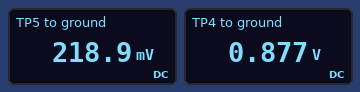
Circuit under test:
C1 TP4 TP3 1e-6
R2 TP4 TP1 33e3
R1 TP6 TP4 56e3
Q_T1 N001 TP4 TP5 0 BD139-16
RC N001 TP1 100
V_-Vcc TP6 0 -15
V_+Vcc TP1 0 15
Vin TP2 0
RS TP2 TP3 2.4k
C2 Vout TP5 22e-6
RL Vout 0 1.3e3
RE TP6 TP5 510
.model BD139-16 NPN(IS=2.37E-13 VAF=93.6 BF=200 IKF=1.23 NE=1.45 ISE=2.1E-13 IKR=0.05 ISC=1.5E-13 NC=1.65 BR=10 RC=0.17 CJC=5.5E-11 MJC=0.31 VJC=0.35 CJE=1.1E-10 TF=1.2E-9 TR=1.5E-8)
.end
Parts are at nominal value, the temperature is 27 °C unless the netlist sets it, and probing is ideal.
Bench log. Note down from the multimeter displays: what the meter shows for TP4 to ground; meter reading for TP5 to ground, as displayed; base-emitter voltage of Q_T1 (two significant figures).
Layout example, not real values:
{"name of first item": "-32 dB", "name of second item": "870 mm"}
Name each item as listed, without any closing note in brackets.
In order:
{"what the meter shows for TP4 to ground": "0.877 V", "meter reading for TP5 to ground, as displayed": "218.9 mV", "base-emitter voltage of Q_T1": "660 mV"}
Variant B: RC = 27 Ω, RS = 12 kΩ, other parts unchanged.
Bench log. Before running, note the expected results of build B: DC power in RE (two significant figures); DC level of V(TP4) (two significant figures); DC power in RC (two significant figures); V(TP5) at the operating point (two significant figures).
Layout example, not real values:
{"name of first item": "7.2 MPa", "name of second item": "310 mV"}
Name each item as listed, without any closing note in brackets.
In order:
{"DC power in RE": "460 mW", "DC level of V(TP4)": "930 mV", "DC power in RC": "24 mW", "V(TP5) at the operating point": "270 mV"}
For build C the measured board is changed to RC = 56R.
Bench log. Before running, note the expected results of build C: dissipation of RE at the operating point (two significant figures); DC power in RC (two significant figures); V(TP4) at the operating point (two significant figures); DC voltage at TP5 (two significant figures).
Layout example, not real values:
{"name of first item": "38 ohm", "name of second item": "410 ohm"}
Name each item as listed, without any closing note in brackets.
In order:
{"dissipation of RE at the operating point": "460 mW", "DC power in RC": "50 mW", "V(TP4) at the operating point": "910 mV", "DC voltage at TP5": "250 mV"}
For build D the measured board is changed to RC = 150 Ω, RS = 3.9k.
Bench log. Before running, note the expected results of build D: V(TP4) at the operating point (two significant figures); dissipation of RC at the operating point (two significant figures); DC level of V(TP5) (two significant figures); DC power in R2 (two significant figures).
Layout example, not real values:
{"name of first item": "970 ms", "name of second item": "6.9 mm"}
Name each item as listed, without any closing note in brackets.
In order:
{"V(TP4) at the operating point": "840 mV", "dissipation of RC at the operating point": "130 mW", "DC level of V(TP5)": "180 mV", "DC power in R2": "6.1 mW"}
